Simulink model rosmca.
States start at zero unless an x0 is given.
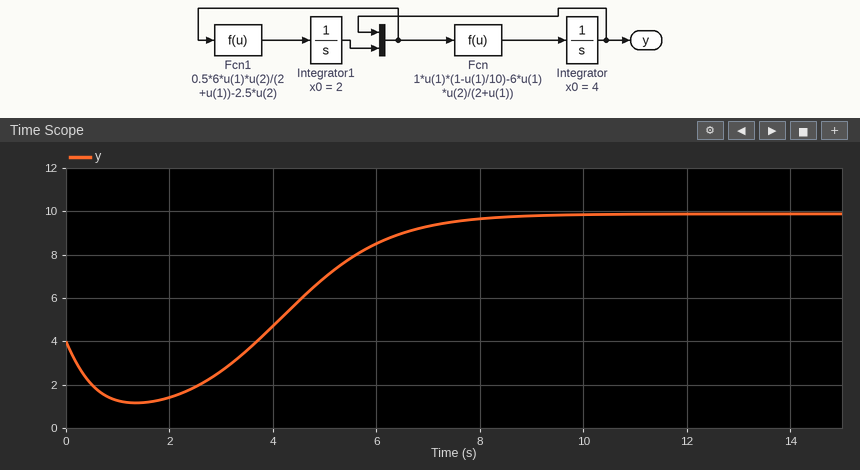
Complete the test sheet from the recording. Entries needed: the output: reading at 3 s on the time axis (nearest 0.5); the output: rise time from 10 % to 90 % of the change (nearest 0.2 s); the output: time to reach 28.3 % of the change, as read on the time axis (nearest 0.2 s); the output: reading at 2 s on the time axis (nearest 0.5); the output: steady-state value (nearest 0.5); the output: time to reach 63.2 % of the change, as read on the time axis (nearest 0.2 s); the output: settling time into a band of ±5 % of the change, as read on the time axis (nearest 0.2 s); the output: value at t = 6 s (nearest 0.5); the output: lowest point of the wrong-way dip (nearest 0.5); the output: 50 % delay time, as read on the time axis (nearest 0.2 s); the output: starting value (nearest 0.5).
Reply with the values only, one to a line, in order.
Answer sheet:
2.5
3.0 s
4.4 s
1.5
10.0
5.4 s
7.8 s
8.5
1.0
5.0 s
4.0
